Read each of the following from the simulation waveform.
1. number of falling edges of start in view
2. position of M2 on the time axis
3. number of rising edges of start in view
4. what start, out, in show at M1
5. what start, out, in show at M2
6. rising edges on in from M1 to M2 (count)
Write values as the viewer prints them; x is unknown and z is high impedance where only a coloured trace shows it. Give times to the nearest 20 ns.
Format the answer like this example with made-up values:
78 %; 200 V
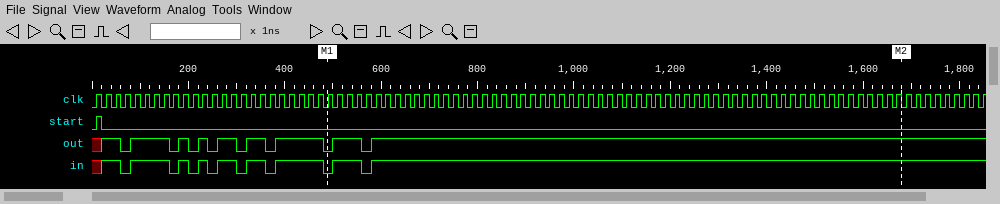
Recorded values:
1; 1680 ns; 1; start=0, out=0, in=0; start=0, out=1, in=1; 2
